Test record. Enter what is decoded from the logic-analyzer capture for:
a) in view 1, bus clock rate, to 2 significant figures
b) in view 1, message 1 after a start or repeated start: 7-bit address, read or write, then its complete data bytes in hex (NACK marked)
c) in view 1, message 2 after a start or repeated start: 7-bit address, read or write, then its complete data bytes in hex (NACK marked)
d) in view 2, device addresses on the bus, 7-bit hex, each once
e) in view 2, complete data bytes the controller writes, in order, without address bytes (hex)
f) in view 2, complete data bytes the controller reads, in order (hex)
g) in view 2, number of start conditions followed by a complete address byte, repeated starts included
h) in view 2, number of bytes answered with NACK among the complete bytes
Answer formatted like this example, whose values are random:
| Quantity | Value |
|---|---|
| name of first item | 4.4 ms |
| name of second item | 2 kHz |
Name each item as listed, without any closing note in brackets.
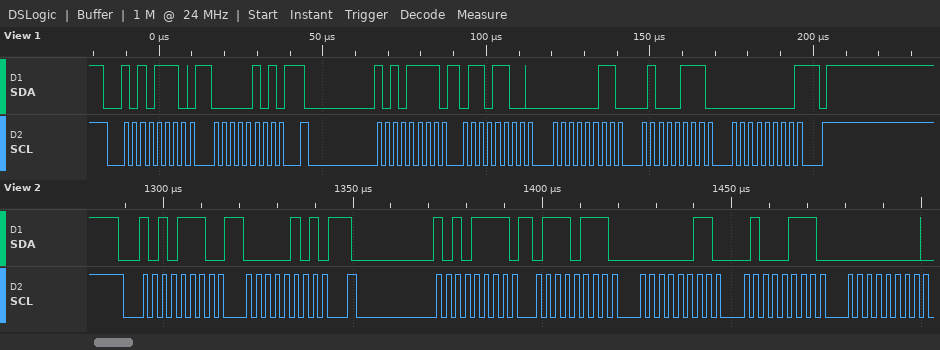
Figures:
| Quantity | Value |
|---|---|
| in view 1, bus clock rate, to 2 significant figures | 400 kHz |
| in view 1, message 1 after a start or repeated start: 7-bit address, read or write, then its complete data bytes in hex | 0x57 write: 05 |
| in view 1, message 2 after a start or repeated start: 7-bit address, read or write, then its complete data bytes in hex | 0x57 read: 6C 03 47 00 NACK |
| in view 2, device addresses on the bus, 7-bit hex, each once | 0x57 |
| in view 2, complete data bytes the controller writes, in order, without address bytes | 05 |
| in view 2, complete data bytes the controller reads, in order | 77 03 47 00 |
| in view 2, number of start conditions followed by a complete address byte, repeated starts included | 2 |
| in view 2, number of bytes answered with NACK among the complete bytes | 0 |
